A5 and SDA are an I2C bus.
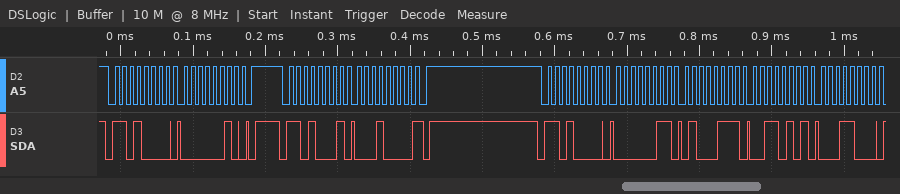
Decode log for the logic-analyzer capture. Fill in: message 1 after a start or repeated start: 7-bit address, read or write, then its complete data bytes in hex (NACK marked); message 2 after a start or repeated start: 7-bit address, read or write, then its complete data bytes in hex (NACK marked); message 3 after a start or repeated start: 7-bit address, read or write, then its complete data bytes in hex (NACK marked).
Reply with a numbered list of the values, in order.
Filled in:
1. 0x68 write: 02
2. 0x68 read: 10 NACK
3. 0x68 write: 03 47 35 18
